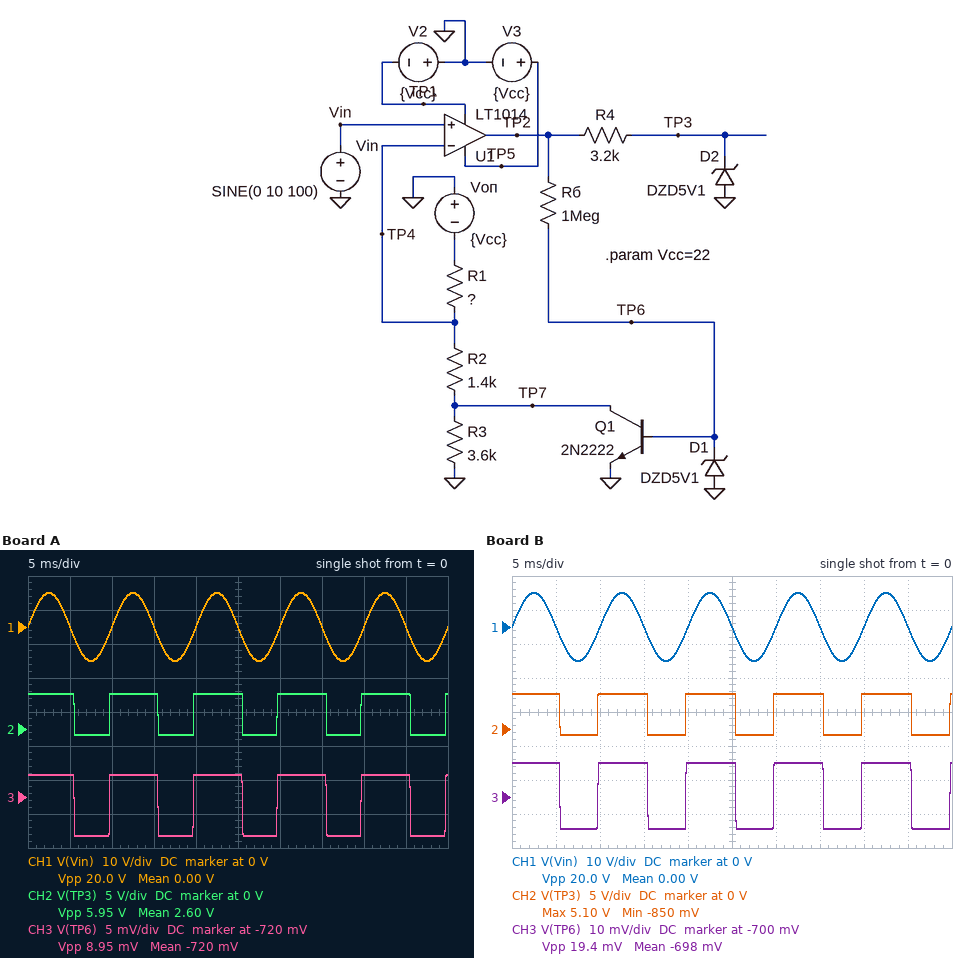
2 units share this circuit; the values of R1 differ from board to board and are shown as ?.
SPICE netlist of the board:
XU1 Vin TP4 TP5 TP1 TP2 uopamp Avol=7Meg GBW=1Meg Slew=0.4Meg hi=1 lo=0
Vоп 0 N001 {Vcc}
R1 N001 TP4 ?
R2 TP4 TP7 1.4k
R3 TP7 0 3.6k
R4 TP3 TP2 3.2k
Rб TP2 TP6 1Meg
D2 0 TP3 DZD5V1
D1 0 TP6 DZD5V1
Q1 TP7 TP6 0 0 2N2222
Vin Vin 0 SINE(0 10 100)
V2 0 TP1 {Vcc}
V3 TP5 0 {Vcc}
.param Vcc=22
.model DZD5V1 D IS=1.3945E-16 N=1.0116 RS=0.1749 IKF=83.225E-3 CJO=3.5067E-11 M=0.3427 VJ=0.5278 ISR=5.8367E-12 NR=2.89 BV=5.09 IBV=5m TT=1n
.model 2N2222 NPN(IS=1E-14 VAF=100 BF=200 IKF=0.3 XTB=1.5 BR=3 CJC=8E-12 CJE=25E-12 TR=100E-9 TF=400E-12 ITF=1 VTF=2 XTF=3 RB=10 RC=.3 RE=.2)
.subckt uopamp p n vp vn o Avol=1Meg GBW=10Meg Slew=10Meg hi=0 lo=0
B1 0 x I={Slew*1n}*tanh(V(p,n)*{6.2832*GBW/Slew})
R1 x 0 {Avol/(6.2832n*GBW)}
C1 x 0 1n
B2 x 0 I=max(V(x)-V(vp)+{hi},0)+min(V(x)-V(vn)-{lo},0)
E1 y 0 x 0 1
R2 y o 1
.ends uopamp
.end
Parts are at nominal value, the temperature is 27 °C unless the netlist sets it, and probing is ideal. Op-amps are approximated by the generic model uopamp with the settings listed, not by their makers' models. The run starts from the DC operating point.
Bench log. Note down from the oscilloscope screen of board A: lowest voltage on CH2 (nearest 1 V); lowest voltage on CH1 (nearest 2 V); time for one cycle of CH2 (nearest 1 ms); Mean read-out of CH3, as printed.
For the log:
-1 V
-10 V
10 ms
-720 mV
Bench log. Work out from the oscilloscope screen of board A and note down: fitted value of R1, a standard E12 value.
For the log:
22 kΩ
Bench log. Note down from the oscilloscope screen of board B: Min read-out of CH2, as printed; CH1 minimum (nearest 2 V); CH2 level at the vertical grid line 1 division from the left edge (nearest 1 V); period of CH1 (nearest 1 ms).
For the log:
-850 mV
-10 V
5 V
10 ms
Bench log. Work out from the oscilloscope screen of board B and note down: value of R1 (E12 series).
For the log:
33 kΩ
